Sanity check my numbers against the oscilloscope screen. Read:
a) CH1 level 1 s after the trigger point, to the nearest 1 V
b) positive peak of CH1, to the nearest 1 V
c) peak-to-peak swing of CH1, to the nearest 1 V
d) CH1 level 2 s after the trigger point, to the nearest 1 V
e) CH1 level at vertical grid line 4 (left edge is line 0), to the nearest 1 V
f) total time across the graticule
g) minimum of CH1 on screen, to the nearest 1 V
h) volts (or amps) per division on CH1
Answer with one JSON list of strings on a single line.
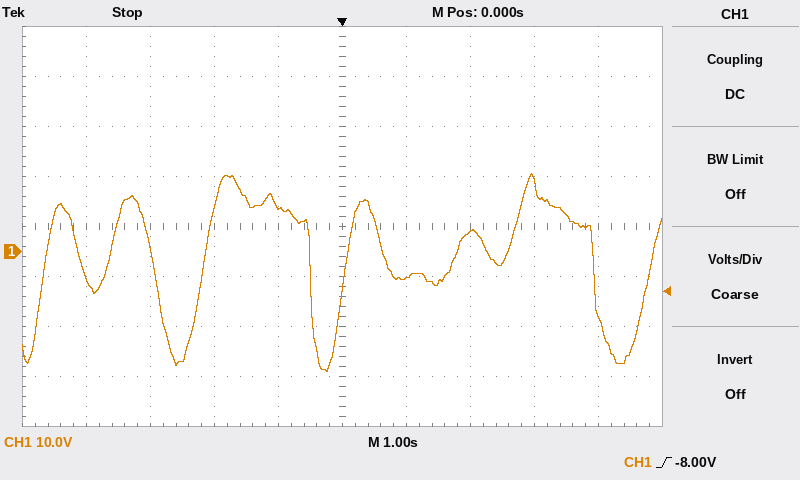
["-5 V", "16 V", "40 V", "4 V", "9 V", "10 s", "-24 V", "10 V"]
